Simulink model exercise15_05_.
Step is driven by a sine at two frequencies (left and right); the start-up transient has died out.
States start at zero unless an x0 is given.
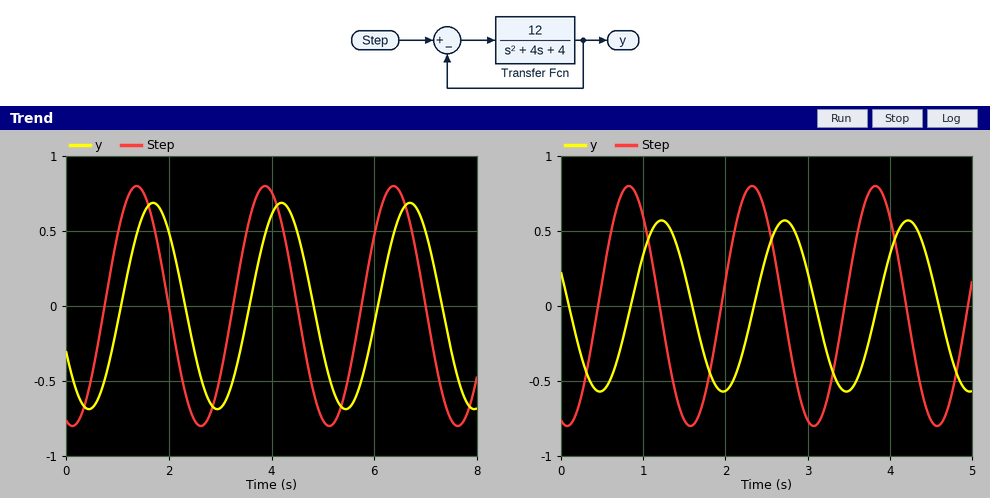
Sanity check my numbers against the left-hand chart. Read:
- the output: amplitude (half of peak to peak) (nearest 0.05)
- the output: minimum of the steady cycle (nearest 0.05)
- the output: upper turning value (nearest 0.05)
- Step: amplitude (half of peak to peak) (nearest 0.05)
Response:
0.70
-0.70
0.70
0.80
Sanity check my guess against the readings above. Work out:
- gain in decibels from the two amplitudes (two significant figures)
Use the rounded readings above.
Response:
-1.2 dB
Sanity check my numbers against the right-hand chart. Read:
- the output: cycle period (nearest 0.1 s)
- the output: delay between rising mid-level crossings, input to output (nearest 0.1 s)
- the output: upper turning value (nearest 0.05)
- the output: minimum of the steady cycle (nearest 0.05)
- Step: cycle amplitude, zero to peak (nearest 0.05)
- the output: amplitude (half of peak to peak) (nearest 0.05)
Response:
1.5 s
0.4 s
0.55
-0.55
0.80
0.55
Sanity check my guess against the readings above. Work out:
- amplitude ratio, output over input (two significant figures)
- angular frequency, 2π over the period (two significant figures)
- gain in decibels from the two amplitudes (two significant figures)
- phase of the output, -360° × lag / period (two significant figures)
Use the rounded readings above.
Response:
0.69
4.2 rad/s
-3.3 dB
-96°
